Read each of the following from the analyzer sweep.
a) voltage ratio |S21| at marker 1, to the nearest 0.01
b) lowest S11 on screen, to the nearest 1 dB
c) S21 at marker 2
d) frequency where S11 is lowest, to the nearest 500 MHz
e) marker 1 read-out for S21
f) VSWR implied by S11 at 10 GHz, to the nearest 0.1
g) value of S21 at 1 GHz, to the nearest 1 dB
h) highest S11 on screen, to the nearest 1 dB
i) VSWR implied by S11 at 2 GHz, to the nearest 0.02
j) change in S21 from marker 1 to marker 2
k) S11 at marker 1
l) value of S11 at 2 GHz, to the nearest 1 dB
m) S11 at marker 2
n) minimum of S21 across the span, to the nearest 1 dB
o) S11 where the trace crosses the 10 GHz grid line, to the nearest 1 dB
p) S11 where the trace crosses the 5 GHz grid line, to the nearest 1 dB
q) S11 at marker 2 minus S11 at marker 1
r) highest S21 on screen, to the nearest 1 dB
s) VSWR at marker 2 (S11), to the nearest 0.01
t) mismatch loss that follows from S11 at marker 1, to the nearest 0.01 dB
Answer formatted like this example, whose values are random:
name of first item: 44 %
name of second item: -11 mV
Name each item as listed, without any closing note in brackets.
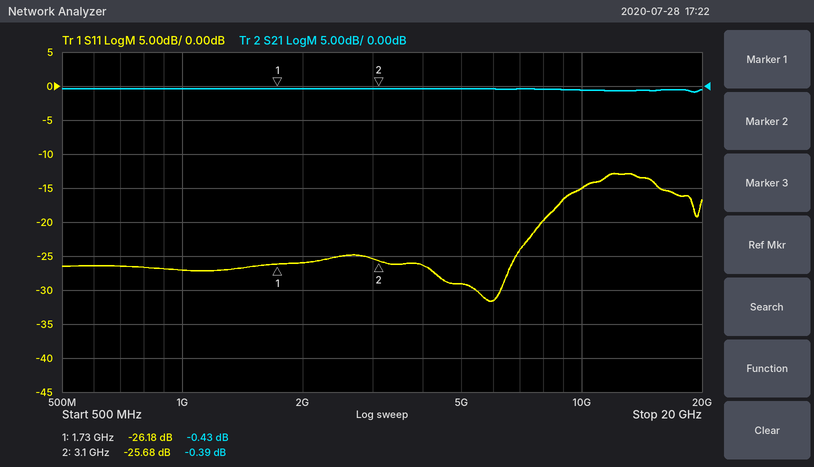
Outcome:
voltage ratio |S21| at marker 1, to the nearest 0.01: 0.95
lowest S11 on screen, to the nearest 1 dB: -32 dB
S21 at marker 2: -0.39 dB
frequency where S11 is lowest, to the nearest 500 MHz: 6.0 GHz
marker 1 read-out for S21: -0.43 dB
VSWR implied by S11 at 10 GHz, to the nearest 0.1: 1.4
value of S21 at 1 GHz, to the nearest 1 dB: 0 dB
highest S11 on screen, to the nearest 1 dB: -13 dB
VSWR implied by S11 at 2 GHz, to the nearest 0.02: 1.10
change in S21 from marker 1 to marker 2: 0.04 dB
S11 at marker 1: -26.18 dB
value of S11 at 2 GHz, to the nearest 1 dB: -26 dB
S11 at marker 2: -25.68 dB
minimum of S21 across the span, to the nearest 1 dB: -1 dB
S11 where the trace crosses the 10 GHz grid line, to the nearest 1 dB: -15 dB
S11 where the trace crosses the 5 GHz grid line, to the nearest 1 dB: -29 dB
S11 at marker 2 minus S11 at marker 1: 0.50 dB
highest S21 on screen, to the nearest 1 dB: 0 dB
VSWR at marker 2 (S11), to the nearest 0.01: 1.11
mismatch loss that follows from S11 at marker 1, to the nearest 0.01 dB: 0.01 dB
